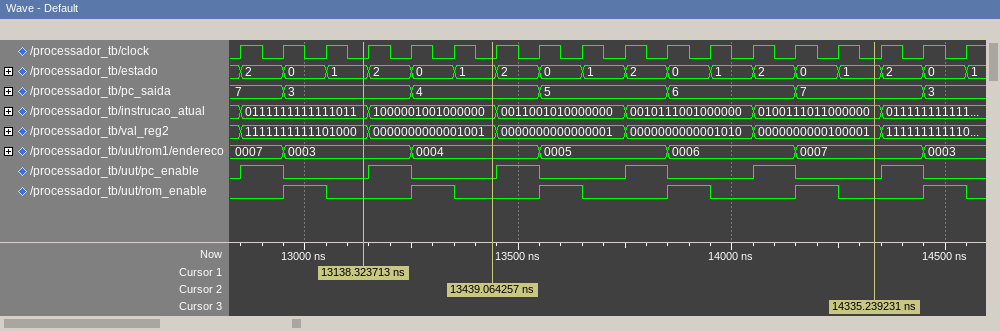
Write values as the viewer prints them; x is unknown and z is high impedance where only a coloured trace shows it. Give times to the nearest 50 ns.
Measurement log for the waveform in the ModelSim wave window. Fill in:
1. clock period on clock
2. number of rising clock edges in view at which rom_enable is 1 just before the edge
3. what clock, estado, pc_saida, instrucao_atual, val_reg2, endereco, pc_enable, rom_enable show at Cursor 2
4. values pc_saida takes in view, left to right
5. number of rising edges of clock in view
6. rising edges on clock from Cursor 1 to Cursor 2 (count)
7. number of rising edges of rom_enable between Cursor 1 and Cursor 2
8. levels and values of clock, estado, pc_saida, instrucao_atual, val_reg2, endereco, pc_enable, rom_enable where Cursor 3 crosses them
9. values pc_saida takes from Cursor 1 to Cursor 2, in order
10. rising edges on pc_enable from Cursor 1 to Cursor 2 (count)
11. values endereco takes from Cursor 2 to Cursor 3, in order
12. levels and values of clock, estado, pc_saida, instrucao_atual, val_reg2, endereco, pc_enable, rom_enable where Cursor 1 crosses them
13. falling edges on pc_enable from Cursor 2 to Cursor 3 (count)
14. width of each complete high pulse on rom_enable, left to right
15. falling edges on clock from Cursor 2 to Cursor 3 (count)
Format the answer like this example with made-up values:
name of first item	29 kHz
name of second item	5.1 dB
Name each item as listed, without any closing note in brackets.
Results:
clock period on clock	100 ns
number of rising clock edges in view at which rom_enable is 1 just before the edge	6
what clock, estado, pc_saida, instrucao_atual, val_reg2, endereco, pc_enable, rom_enable show at Cursor 2	clock=0, estado=1, pc_saida=4, instrucao_atual=1000001001000000, val_reg2=0000000000001001, endereco=0004, pc_enable=0, rom_enable=0
values pc_saida takes in view, left to right	7, 3, 4, 5, 6, 7, 3
number of rising edges of clock in view	18
rising edges on clock from Cursor 1 to Cursor 2	3
number of rising edges of rom_enable between Cursor 1 and Cursor 2	1
levels and values of clock, estado, pc_saida, instrucao_atual, val_reg2, endereco, pc_enable, rom_enable where Cursor 3 crosses them	clock=0, estado=1, pc_saida=7, instrucao_atual=0100111011000000, val_reg2=0000000000100001, endereco=0007, pc_enable=0, rom_enable=0
values pc_saida takes from Cursor 1 to Cursor 2, in order	3, 4
rising edges on pc_enable from Cursor 1 to Cursor 2	1
values endereco takes from Cursor 2 to Cursor 3, in order	0004, 0005, 0006, 0007
levels and values of clock, estado, pc_saida, instrucao_atual, val_reg2, endereco, pc_enable, rom_enable where Cursor 1 crosses them	clock=0, estado=1, pc_saida=3, instrucao_atual=0111111111111011, val_reg2=1111111111101000, endereco=0003, pc_enable=0, rom_enable=0
falling edges on pc_enable from Cursor 2 to Cursor 3	3
width of each complete high pulse on rom_enable, left to right	100 ns, 100 ns, 100 ns, 100 ns, 100 ns, 100 ns
falling edges on clock from Cursor 2 to Cursor 3	9
